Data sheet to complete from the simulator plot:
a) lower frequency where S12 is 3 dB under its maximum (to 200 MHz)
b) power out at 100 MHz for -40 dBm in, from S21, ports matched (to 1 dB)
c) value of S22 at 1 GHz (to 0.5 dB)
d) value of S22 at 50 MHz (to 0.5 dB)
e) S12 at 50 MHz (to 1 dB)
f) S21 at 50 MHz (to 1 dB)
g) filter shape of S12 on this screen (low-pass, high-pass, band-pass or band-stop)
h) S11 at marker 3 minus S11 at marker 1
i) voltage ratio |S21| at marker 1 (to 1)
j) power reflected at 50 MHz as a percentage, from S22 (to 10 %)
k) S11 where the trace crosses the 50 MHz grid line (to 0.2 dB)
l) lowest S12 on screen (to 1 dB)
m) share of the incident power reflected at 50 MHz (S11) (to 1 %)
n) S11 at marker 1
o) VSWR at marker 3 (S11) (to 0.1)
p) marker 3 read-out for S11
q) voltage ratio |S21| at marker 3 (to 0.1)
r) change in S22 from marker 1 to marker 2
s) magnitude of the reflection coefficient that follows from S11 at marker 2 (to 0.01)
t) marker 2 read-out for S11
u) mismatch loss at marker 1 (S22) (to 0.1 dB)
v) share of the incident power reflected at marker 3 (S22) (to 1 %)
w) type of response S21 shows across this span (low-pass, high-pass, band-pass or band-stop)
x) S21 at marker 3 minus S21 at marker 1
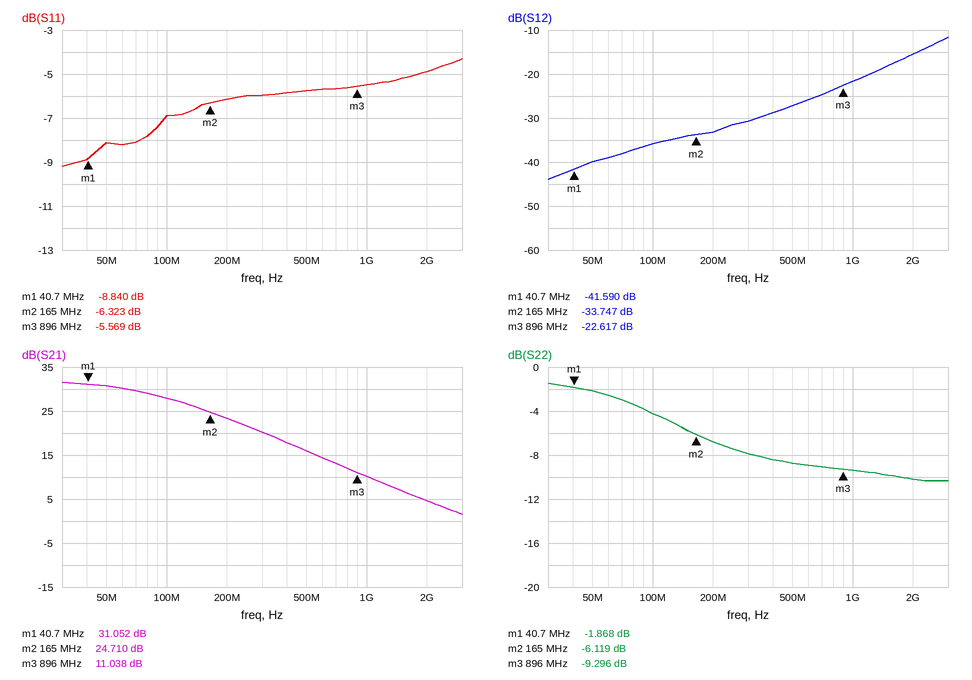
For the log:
2.2 GHz
-12 dBm
-9.5 dB
-2.0 dB
-40 dB
31 dB
high-pass
3.271 dB
36
60 %
-8.2 dB
-44 dB
15 %
-8.840 dB
3.2
-5.569 dB
3.6
-4.251 dB
0.48
-6.323 dB
4.6 dB
12 %
low-pass
-20.014 dB
